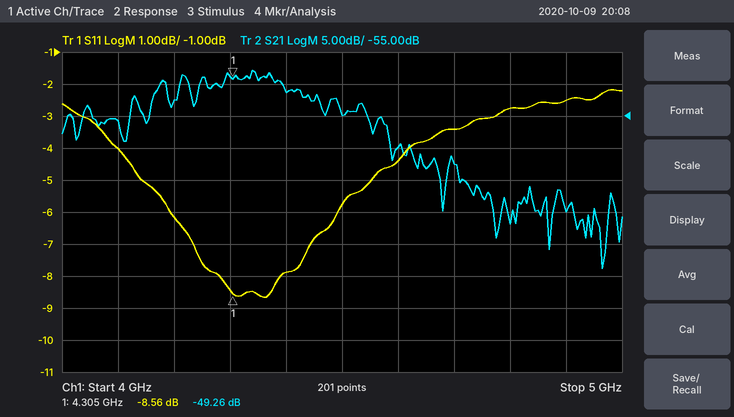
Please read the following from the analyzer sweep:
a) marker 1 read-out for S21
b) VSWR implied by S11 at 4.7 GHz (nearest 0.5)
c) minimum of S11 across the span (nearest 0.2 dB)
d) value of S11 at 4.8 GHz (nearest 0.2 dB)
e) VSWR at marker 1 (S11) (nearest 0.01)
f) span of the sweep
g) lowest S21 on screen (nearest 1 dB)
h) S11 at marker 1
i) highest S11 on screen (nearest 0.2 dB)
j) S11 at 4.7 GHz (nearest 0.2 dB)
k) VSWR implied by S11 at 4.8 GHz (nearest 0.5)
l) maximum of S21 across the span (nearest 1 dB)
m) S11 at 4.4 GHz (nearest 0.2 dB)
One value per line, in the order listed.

-49.26 dB
5.0
-8.6 dB
-2.8 dB
2.19
1 GHz
-79 dB
-8.56 dB
-2.2 dB
-3.4 dB
6.5
-48 dB
-7.8 dB
